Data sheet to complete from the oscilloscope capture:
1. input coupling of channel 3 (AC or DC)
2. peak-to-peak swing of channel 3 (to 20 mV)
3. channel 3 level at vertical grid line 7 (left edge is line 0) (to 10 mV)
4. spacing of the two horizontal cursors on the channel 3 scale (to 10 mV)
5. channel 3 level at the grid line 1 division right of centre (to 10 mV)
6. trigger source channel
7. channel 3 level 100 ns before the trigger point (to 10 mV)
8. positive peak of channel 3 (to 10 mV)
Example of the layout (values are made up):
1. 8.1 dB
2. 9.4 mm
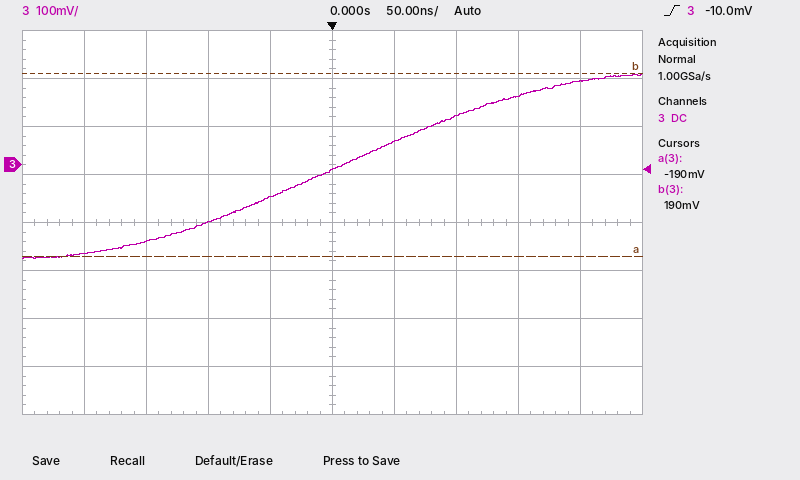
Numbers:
1. DC
2. 380 mV
3. 100 mV
4. 380 mV
5. 50 mV
6. channel 3
7. -120 mV
8. 190 mV
